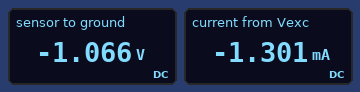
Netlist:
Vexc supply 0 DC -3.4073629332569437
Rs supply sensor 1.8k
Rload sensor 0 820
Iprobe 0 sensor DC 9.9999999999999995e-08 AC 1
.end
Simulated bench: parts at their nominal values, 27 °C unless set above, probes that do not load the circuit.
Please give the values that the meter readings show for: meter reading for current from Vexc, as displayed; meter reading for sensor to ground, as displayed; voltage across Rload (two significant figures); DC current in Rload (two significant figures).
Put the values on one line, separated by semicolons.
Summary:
-1.301 mA; -1.066 V; 1.1 V; 1.3 mA
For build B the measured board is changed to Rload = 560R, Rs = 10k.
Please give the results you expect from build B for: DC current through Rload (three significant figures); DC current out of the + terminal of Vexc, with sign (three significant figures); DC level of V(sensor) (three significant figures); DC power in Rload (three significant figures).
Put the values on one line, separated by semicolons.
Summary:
323 µA; -323 µA; -181 mV; 58.3 µW
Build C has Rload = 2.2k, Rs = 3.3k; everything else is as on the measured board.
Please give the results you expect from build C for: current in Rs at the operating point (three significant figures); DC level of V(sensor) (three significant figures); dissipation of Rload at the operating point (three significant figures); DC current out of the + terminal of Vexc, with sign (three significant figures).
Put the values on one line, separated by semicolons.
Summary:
620 µA; -1.36 V; 844 µW; -620 µA
